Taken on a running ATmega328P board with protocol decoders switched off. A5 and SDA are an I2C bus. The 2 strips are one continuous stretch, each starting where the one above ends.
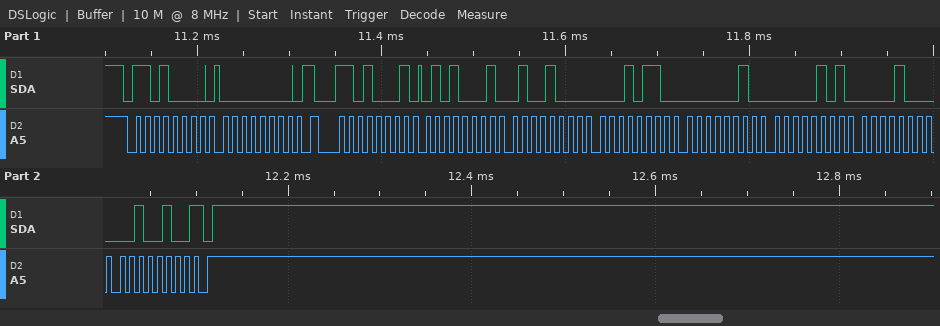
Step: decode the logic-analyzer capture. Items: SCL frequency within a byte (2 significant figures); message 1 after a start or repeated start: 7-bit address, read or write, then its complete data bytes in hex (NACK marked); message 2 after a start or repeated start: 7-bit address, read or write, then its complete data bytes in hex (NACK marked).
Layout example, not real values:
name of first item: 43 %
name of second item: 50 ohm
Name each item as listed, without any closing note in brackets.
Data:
SCL frequency within a byte: 100 kHz
message 1 after a start or repeated start: 7-bit address, read or write, then its complete data bytes in hex: 0x68 write: 00
message 2 after a start or repeated start: 7-bit address, read or write, then its complete data bytes in hex: 0x68 read: 51 48 16 02 05 08 24 NACK
